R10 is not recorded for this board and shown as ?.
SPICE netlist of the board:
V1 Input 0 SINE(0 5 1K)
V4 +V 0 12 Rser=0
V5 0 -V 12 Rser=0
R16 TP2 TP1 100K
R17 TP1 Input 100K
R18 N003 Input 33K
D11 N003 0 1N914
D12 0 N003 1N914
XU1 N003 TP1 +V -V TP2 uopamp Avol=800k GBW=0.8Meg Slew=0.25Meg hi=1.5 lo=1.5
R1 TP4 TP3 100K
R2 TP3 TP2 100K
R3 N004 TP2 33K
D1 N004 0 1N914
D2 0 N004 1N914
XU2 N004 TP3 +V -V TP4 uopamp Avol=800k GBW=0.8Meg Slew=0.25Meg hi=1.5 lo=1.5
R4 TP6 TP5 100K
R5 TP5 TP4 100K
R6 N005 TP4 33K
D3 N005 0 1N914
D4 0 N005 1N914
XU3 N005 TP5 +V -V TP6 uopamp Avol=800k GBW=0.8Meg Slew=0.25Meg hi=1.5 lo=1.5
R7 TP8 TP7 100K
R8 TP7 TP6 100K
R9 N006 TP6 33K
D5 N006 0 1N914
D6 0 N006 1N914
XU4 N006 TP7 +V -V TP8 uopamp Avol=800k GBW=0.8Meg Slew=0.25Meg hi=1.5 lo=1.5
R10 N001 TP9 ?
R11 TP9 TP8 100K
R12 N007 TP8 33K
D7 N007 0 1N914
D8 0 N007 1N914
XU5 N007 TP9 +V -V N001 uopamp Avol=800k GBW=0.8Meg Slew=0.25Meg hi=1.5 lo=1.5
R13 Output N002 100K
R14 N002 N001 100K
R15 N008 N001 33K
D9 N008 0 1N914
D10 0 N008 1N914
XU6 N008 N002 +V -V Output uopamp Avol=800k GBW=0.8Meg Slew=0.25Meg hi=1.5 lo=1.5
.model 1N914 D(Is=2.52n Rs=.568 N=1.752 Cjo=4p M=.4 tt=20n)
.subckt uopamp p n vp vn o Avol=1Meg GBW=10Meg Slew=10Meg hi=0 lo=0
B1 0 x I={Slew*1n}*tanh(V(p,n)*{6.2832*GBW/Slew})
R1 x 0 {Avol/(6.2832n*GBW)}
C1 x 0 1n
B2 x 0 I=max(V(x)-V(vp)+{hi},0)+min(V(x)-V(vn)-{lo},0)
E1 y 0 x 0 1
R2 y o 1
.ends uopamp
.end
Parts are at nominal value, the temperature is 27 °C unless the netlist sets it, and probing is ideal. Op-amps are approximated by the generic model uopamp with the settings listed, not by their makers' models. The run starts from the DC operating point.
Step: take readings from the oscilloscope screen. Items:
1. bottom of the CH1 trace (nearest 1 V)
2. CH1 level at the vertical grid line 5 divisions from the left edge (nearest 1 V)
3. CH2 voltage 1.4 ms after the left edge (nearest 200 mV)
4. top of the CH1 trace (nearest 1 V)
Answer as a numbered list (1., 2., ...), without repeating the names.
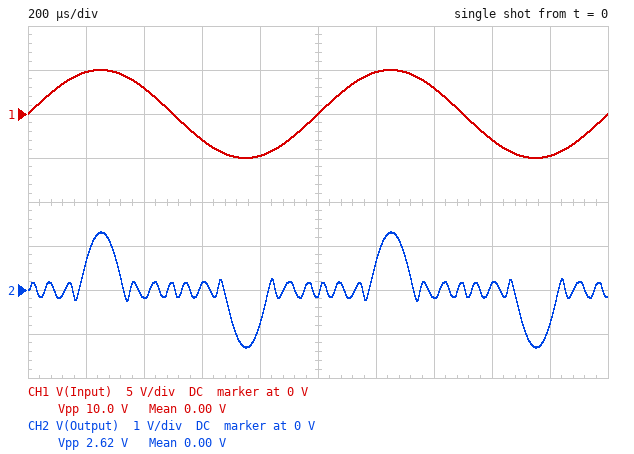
1. -5 V
2. 0 V
3. -200 mV
4. 5 V
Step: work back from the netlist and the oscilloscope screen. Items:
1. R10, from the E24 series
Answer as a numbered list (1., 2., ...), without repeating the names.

1. 330 kΩ
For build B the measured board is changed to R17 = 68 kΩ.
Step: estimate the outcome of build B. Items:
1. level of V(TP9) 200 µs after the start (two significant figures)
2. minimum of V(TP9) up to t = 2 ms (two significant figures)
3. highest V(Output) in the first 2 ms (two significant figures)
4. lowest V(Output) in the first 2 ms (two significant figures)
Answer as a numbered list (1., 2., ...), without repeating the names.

1. 470 mV
2. -470 mV
3. 7.4 V
4. -7.4 V
